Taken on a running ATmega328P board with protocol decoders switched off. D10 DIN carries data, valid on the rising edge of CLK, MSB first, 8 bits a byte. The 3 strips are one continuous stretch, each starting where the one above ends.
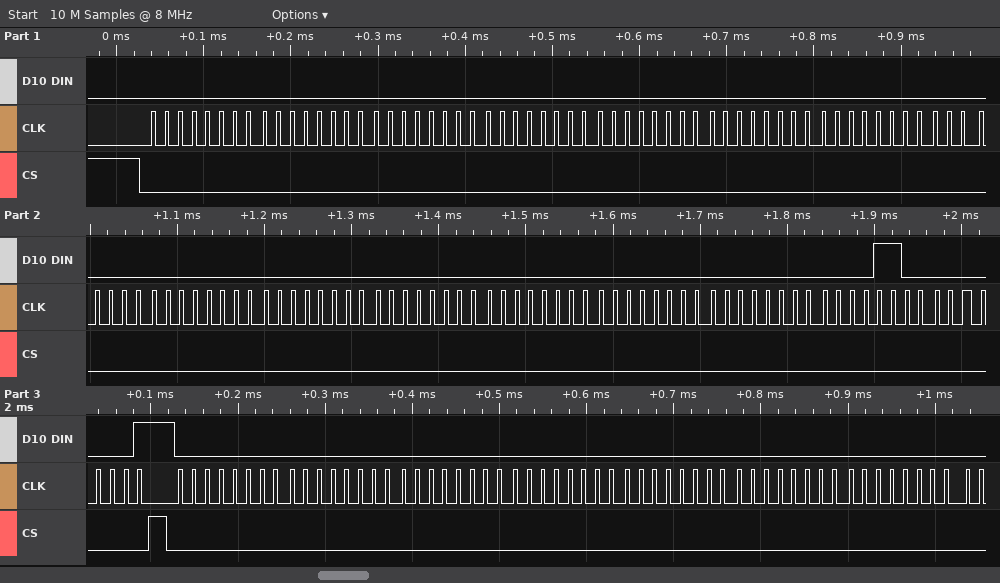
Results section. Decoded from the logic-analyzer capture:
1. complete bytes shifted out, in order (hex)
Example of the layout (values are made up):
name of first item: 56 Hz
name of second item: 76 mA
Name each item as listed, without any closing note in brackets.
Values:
complete bytes shifted out, in order: 00 00 00 00 00 00 00 00 00 00 00 00 00 00 0C 01 00 00 00 00 00 00 00
